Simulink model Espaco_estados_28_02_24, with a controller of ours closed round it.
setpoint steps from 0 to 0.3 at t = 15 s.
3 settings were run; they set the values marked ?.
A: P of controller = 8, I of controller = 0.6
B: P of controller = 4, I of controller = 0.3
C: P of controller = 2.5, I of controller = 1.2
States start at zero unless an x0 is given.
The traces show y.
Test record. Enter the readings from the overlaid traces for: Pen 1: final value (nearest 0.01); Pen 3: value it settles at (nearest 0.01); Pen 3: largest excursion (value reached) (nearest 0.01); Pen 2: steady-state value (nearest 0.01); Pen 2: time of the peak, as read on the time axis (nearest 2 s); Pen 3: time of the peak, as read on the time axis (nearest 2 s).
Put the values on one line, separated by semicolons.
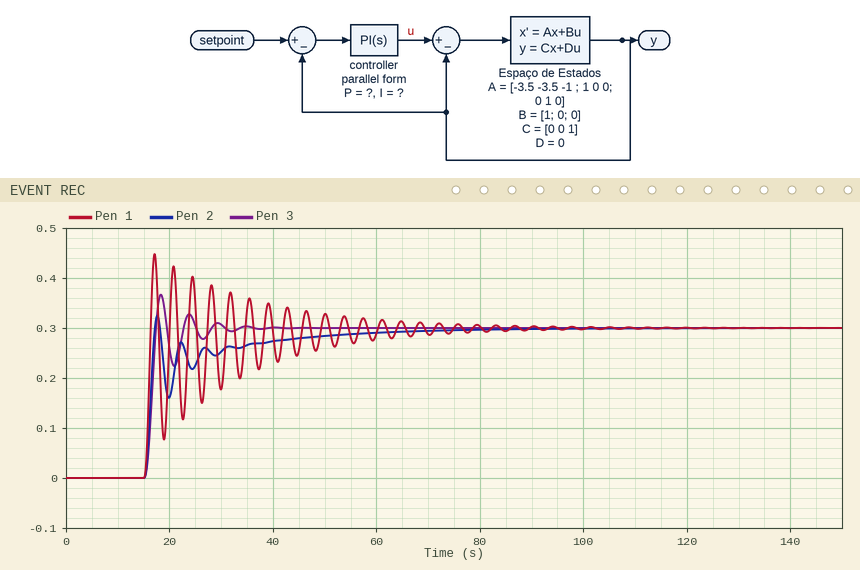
0.30; 0.30; 0.37; 0.30; 18 s; 18 s
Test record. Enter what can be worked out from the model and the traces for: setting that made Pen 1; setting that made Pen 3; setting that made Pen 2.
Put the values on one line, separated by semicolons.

A; C; B
